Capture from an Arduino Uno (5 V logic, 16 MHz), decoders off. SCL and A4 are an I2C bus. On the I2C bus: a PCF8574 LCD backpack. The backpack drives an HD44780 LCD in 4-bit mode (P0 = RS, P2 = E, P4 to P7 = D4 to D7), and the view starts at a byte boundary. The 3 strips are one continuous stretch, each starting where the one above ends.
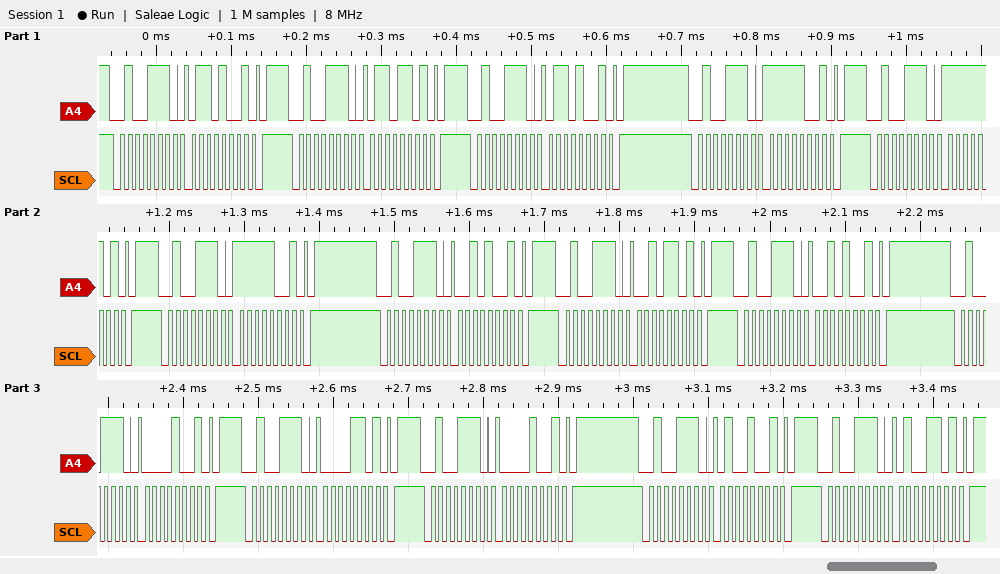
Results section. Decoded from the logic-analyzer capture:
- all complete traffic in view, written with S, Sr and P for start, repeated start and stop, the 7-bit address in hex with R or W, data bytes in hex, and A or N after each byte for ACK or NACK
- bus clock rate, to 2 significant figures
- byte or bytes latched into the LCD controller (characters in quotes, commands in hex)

S 27W A 69 A P S 27W A 6D A P S 27W A 69 A P S 27W A F9 A P S 27W A FD A P S 27W A F9 A P S 27W A 29 A P S 27W A 2D A P S 27W A 29 A P S 27W A 09 A P S 27W A 0D A P S 27W A 09 A P S 27W A 49 A P S 27W A 4D A P
100 kHz
'o' ' '
